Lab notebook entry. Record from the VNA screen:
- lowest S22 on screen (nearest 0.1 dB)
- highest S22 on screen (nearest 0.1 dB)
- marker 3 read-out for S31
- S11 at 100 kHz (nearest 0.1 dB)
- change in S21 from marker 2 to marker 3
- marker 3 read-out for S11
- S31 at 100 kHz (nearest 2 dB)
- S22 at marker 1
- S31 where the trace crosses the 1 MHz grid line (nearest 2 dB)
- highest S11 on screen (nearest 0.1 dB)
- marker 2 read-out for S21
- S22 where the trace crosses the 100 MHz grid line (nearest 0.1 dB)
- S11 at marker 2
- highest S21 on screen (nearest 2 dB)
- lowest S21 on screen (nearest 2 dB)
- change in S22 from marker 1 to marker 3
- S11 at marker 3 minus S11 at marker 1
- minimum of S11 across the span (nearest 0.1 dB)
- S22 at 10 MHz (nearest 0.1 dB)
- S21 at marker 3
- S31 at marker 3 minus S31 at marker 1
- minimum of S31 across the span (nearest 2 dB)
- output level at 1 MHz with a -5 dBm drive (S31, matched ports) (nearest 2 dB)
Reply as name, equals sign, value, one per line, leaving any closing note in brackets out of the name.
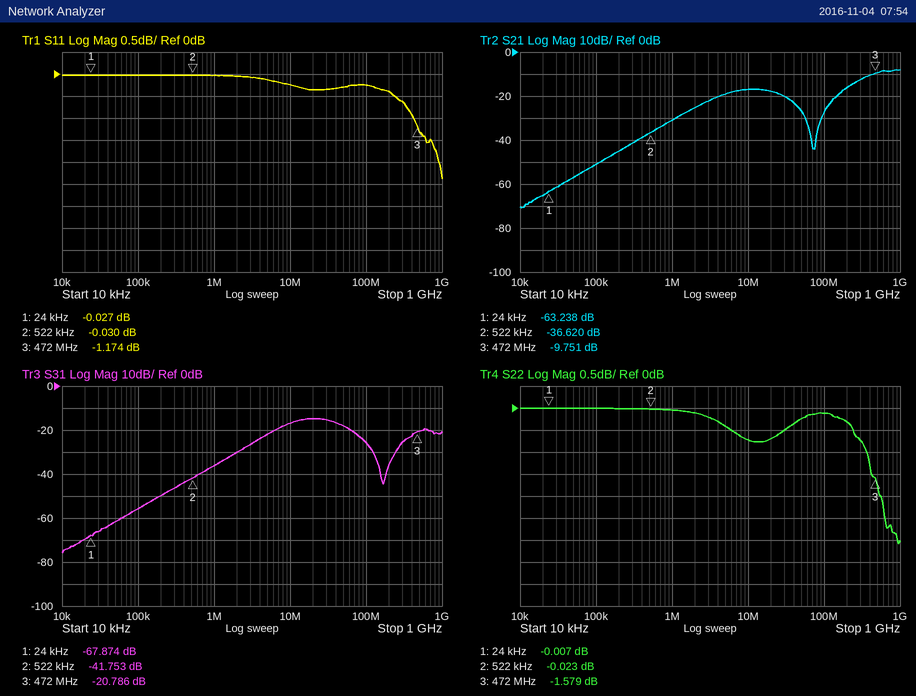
lowest S22 on screen = -3.1 dB
highest S22 on screen = 0.0 dB
marker 3 read-out for S31 = -20.786 dB
S11 at 100 kHz = 0.0 dB
change in S21 from marker 2 to marker 3 = 26.869 dB
marker 3 read-out for S11 = -1.174 dB
S31 at 100 kHz = -56 dB
S22 at marker 1 = -0.007 dB
S31 where the trace crosses the 1 MHz grid line = -36 dB
highest S11 on screen = 0.0 dB
marker 2 read-out for S21 = -36.620 dB
S22 where the trace crosses the 100 MHz grid line = -0.1 dB
S11 at marker 2 = -0.030 dB
highest S21 on screen = -8 dB
lowest S21 on screen = -70 dB
change in S22 from marker 1 to marker 3 = -1.572 dB
S11 at marker 3 minus S11 at marker 1 = -1.147 dB
minimum of S11 across the span = -2.4 dB
S22 at 10 MHz = -0.7 dB
S21 at marker 3 = -9.751 dB
S31 at marker 3 minus S31 at marker 1 = 47.088 dB
minimum of S31 across the span = -76 dB
output level at 1 MHz with a -5 dBm drive (S31, matched ports) = -42 dBm
